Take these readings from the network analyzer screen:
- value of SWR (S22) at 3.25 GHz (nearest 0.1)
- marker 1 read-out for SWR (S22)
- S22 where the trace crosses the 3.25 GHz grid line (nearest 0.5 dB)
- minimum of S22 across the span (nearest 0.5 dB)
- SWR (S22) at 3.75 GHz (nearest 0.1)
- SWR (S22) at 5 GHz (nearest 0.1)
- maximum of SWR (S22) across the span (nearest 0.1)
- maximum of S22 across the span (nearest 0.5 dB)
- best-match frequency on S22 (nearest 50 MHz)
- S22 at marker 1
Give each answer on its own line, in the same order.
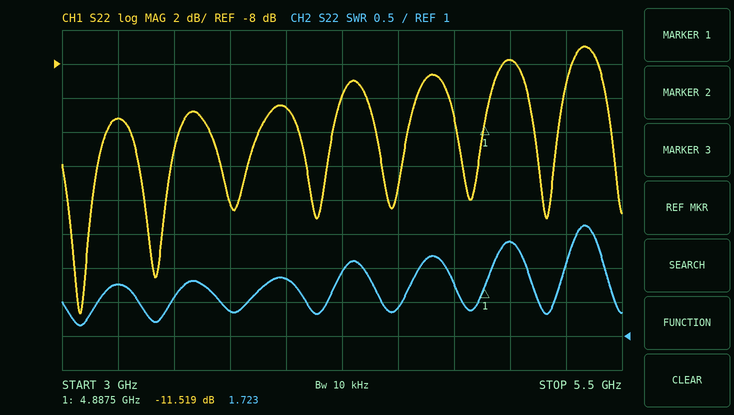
1.8
1.723
-11.0 dB
-22.5 dB
1.4
2.4
2.6
-7.0 dB
3.10 GHz
-11.519 dB
